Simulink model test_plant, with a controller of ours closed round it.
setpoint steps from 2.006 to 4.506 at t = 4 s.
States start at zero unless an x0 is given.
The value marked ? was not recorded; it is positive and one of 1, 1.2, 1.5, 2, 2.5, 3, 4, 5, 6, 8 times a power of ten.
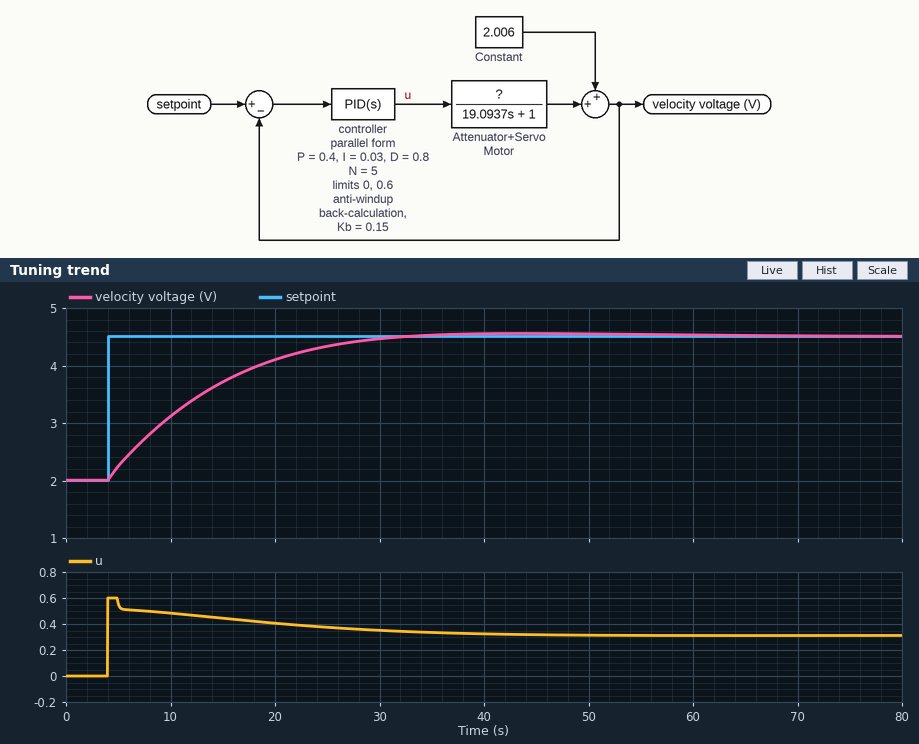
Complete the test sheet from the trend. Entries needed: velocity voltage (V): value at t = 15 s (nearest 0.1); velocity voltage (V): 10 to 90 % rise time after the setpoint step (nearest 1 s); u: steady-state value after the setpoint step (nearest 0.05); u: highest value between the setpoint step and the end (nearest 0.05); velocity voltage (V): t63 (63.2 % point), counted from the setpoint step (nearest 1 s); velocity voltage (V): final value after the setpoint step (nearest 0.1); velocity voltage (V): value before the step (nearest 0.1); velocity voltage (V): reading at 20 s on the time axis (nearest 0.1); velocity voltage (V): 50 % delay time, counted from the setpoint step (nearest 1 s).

3.7
18 s
0.30
0.60
10 s
4.5
2.0
4.1
7 s
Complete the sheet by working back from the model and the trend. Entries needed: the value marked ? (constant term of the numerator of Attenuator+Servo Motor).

8
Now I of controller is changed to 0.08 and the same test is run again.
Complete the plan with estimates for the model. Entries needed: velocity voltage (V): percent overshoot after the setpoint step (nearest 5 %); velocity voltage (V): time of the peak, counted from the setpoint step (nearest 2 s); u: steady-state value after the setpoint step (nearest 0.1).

15 %
22 s
0.3
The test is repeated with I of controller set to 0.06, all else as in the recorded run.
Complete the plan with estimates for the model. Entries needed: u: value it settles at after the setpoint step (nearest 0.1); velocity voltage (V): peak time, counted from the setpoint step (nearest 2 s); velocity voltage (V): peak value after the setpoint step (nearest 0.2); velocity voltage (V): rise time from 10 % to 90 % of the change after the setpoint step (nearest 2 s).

0.3
24 s
4.8
12 s
